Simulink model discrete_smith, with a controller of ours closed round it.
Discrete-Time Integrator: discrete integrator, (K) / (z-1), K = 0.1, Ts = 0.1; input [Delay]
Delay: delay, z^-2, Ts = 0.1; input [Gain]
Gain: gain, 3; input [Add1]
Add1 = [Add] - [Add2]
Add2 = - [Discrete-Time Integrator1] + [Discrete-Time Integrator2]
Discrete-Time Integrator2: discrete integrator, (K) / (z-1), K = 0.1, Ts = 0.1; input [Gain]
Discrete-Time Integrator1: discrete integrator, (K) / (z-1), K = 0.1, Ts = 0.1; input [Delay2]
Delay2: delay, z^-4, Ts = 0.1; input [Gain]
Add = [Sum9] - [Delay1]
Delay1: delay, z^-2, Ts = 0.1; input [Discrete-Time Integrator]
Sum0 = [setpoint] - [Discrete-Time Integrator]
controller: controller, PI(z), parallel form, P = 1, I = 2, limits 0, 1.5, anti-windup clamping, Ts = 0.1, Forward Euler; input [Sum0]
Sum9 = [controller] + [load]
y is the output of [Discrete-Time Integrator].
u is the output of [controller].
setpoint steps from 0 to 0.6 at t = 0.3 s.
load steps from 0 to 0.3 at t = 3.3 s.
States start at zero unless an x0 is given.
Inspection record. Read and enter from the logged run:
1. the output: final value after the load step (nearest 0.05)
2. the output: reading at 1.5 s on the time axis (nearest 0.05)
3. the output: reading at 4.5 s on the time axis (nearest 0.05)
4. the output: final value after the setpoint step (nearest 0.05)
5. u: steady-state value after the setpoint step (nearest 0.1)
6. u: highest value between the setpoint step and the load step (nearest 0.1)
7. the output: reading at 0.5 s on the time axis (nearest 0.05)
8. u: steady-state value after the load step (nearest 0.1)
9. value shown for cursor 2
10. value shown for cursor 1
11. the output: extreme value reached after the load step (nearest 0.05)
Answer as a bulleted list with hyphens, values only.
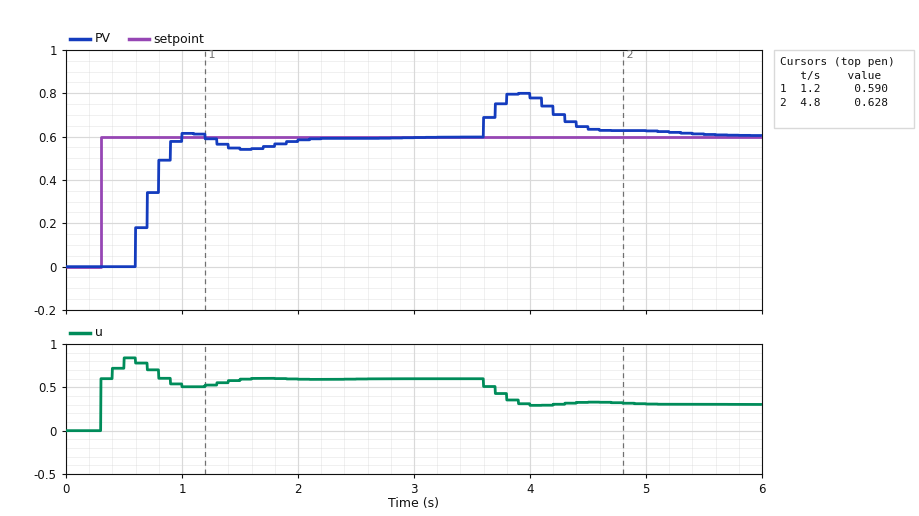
- 0.60
- 0.55
- 0.65
- 0.60
- 0.6
- 0.8
- 0.00
- 0.3
- 0.628
- 0.590
- 0.80
